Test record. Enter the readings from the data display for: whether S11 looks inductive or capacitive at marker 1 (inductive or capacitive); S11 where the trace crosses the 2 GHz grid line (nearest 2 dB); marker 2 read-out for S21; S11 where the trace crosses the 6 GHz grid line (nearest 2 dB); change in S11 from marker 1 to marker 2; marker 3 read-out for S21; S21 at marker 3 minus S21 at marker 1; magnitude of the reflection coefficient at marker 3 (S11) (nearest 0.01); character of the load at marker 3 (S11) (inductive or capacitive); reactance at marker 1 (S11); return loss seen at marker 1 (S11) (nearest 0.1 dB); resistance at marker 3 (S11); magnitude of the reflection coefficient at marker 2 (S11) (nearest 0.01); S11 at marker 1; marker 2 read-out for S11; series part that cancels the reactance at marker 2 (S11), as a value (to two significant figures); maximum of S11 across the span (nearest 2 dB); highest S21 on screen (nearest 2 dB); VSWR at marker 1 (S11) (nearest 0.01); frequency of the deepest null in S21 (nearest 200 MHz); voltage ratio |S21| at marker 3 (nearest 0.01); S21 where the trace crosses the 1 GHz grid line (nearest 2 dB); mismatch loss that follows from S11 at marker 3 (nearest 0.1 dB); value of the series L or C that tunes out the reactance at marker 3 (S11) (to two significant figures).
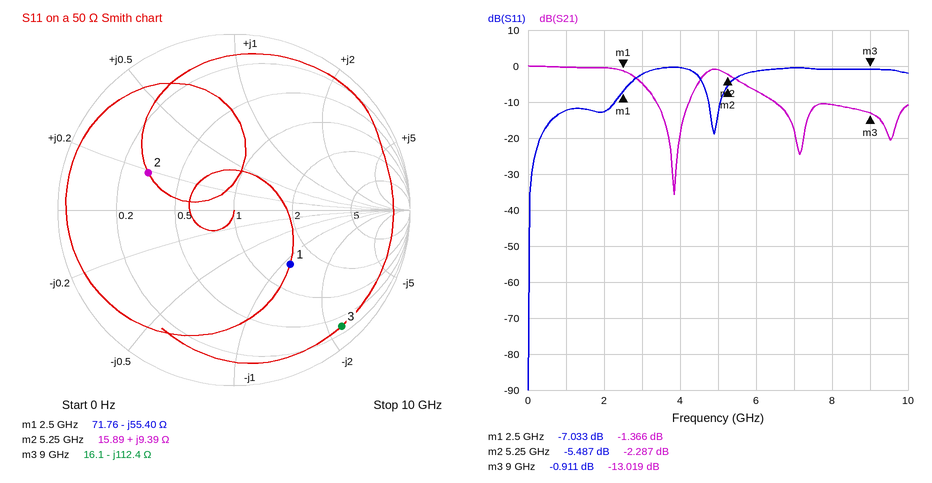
capacitive
-12 dB
-2.287 dB
-2 dB
1.546 dB
-13.019 dB
-11.653 dB
0.90
capacitive
-55.40 Ω
7.0 dB
16.1 Ω
0.53
-7.033 dB
-5.487 dB
3.2 pF
0 dB
0 dB
2.60
3.8 GHz
0.22
0 dB
7.2 dB
2.0 nH
